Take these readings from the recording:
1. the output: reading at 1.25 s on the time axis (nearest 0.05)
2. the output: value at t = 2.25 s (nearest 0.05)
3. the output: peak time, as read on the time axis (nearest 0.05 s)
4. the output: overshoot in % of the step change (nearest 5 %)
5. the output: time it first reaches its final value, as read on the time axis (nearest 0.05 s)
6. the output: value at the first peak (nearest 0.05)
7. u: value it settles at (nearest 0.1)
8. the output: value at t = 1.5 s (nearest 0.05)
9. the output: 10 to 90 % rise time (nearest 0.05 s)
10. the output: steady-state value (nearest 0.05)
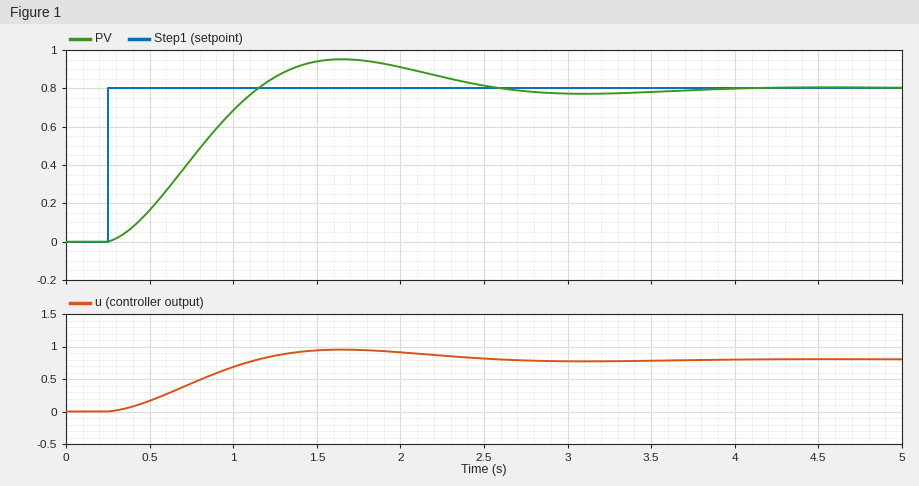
0.85
0.85
1.65 s
20 %
1.15 s
0.95
0.8
0.95
0.65 s
0.80
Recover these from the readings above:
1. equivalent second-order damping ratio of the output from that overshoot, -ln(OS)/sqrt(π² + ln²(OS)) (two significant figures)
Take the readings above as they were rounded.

0.46
